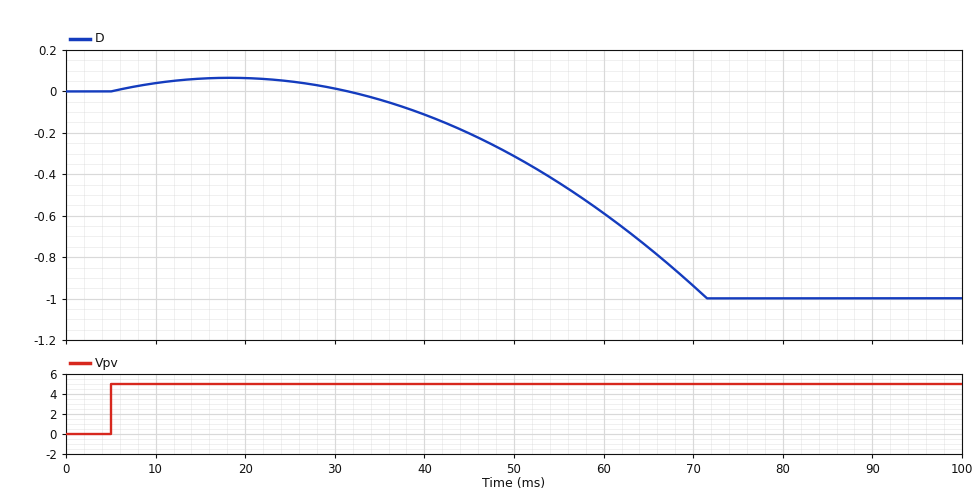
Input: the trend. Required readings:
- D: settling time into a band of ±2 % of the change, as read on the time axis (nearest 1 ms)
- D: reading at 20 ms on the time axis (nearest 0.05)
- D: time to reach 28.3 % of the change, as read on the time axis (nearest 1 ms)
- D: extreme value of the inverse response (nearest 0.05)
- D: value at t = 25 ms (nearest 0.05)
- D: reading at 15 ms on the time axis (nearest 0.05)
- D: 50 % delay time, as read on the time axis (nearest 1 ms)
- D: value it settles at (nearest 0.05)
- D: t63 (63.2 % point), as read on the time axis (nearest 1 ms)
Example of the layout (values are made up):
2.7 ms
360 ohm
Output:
71 ms
0.05
49 ms
0.05
0.05
0.05
57 ms
-1.00
61 ms
